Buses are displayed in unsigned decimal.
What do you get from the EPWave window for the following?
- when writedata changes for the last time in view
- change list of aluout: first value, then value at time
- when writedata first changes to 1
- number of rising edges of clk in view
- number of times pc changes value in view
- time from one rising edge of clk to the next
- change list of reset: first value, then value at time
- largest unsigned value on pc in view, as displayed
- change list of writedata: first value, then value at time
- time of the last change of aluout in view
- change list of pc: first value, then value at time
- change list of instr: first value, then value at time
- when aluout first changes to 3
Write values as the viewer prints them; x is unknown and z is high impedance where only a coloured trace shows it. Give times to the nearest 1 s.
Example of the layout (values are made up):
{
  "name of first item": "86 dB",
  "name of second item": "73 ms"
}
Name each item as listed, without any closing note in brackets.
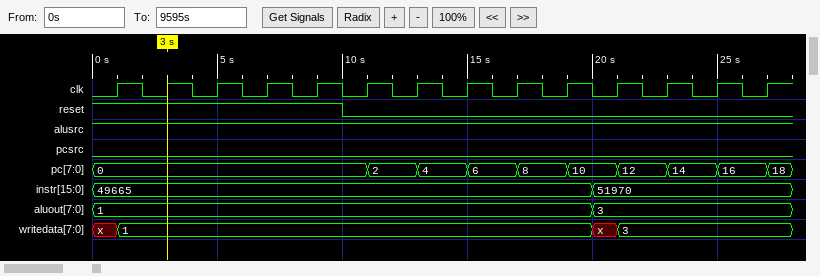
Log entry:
{
  "when writedata changes for the last time in view": "21 s",
  "change list of aluout: first value, then value at time": "1, 3 at 20 s",
  "when writedata first changes to 1": "1 s",
  "number of rising edges of clk in view": "14",
  "number of times pc changes value in view": "9",
  "time from one rising edge of clk to the next": "2 s",
  "change list of reset: first value, then value at time": "1, 0 at 10 s",
  "largest unsigned value on pc in view, as displayed": "18",
  "change list of writedata: first value, then value at time": "x, 1 at 1 s, x at 20 s, 3 at 21 s",
  "time of the last change of aluout in view": "20 s",
  "change list of pc: first value, then value at time": "0, 2 at 11 s, 4 at 13 s, 6 at 15 s, 8 at 17 s, 10 at 19 s, 12 at 21 s, 14 at 23 s, 16 at 25 s, 18 at 27 s",
  "change list of instr: first value, then value at time": "49665, 51970 at 20 s",
  "when aluout first changes to 3": "20 s"
}
